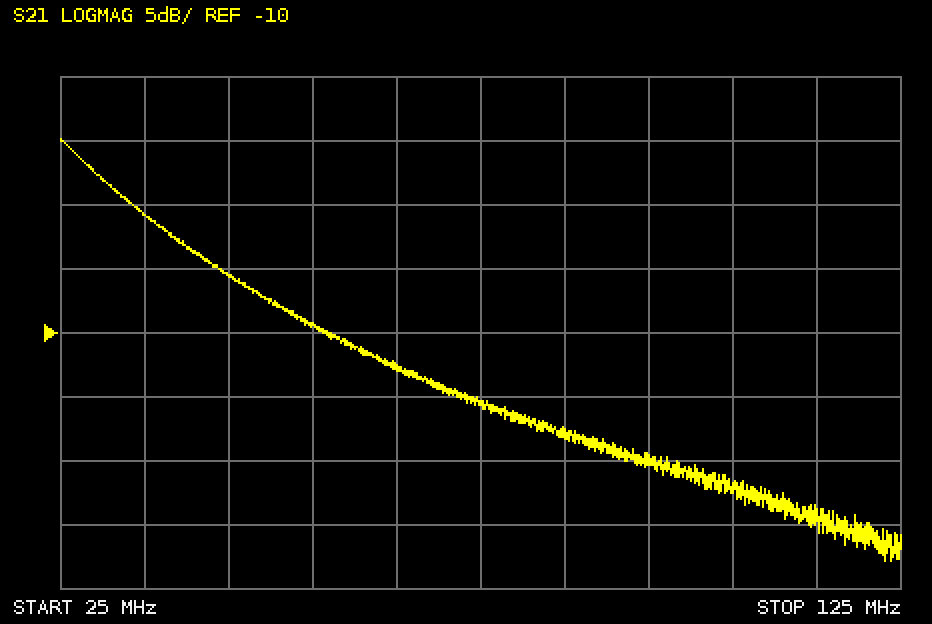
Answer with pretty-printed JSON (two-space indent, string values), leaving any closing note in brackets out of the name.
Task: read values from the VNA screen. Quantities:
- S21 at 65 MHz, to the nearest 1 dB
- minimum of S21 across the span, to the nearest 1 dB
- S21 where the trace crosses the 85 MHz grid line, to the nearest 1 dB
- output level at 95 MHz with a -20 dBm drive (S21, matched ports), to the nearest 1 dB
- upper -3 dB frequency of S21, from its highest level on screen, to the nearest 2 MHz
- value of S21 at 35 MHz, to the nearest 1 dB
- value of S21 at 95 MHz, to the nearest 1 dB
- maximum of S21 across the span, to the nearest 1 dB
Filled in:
{
  "S21 at 65 MHz, to the nearest 1 dB": "-13 dB",
  "minimum of S21 across the span, to the nearest 1 dB": "-28 dB",
  "S21 where the trace crosses the 85 MHz grid line, to the nearest 1 dB": "-18 dB",
  "output level at 95 MHz with a -20 dBm drive (S21, matched ports), to the nearest 1 dB": "-40 dBm",
  "upper -3 dB frequency of S21, from its highest level on screen, to the nearest 2 MHz": "30 MHz",
  "value of S21 at 35 MHz, to the nearest 1 dB": "-1 dB",
  "value of S21 at 95 MHz, to the nearest 1 dB": "-20 dB",
  "maximum of S21 across the span, to the nearest 1 dB": "5 dB"
}
